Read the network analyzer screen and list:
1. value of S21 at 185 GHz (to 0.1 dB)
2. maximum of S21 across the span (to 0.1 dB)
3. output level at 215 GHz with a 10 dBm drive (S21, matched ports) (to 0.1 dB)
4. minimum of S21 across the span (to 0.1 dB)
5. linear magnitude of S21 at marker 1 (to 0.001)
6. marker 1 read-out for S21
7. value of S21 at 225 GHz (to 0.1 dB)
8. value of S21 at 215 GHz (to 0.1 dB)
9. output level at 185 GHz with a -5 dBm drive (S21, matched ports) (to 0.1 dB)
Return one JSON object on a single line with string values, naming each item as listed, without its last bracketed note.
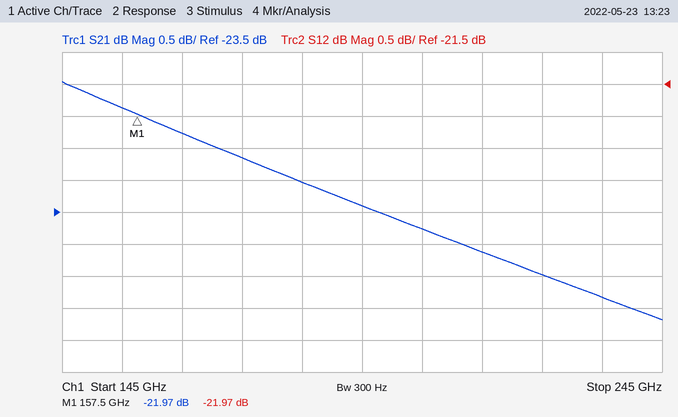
{"value of S21 at 185 GHz": "-23.0 dB", "maximum of S21 across the span": "-21.5 dB", "output level at 215 GHz with a 10 dBm drive (S21, matched ports)": "-14.1 dBm", "minimum of S21 across the span": "-25.2 dB", "linear magnitude of S21 at marker 1": "0.080", "marker 1 read-out for S21": "-21.97 dB", "value of S21 at 225 GHz": "-24.5 dB", "value of S21 at 215 GHz": "-24.1 dB", "output level at 185 GHz with a -5 dBm drive (S21, matched ports)": "-28.0 dBm"}
